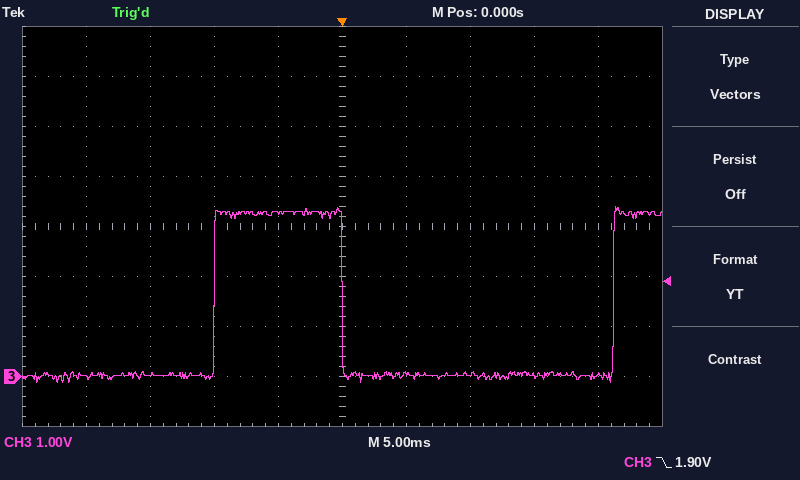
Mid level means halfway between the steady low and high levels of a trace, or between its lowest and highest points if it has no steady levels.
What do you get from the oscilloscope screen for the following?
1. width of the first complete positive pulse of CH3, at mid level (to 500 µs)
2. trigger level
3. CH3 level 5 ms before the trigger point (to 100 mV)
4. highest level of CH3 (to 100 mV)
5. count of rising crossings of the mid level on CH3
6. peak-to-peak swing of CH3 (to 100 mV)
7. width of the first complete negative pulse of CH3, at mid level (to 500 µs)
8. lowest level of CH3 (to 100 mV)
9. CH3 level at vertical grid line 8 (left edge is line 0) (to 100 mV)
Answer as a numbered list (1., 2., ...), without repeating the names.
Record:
1. 10.0 ms
2. 1.90 V
3. 3.3 V
4. 3.4 V
5. 2
6. 3.5 V
7. 21.0 ms
8. -100 mV
9. 0.0 V
